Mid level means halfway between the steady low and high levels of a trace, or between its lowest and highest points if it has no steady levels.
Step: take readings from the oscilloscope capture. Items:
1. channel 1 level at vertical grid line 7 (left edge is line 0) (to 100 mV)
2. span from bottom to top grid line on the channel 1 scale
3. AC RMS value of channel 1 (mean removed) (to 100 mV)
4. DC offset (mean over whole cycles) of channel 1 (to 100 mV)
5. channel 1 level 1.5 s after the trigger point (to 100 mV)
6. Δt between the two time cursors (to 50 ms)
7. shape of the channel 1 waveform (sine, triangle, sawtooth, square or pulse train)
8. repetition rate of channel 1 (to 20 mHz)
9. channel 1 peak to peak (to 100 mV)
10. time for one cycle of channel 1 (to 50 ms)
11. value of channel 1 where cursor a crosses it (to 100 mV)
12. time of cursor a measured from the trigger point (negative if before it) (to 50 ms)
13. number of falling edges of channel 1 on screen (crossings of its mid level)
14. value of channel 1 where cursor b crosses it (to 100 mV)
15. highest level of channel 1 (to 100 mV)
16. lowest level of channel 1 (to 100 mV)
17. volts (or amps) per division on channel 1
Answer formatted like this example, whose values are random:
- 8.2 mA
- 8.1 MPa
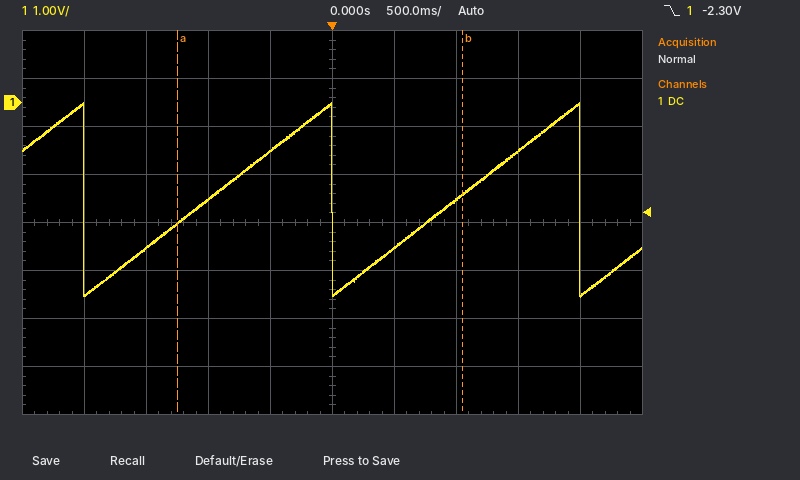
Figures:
- -2.0 V
- 8 V
- 1.2 V
- -2.0 V
- -1.0 V
- 2.30 s
- sawtooth
- 500 mHz
- 4.1 V
- 2.00 s
- -2.5 V
- -1.25 s
- 3
- -1.9 V
- 0.0 V
- -4.1 V
- 1 V
